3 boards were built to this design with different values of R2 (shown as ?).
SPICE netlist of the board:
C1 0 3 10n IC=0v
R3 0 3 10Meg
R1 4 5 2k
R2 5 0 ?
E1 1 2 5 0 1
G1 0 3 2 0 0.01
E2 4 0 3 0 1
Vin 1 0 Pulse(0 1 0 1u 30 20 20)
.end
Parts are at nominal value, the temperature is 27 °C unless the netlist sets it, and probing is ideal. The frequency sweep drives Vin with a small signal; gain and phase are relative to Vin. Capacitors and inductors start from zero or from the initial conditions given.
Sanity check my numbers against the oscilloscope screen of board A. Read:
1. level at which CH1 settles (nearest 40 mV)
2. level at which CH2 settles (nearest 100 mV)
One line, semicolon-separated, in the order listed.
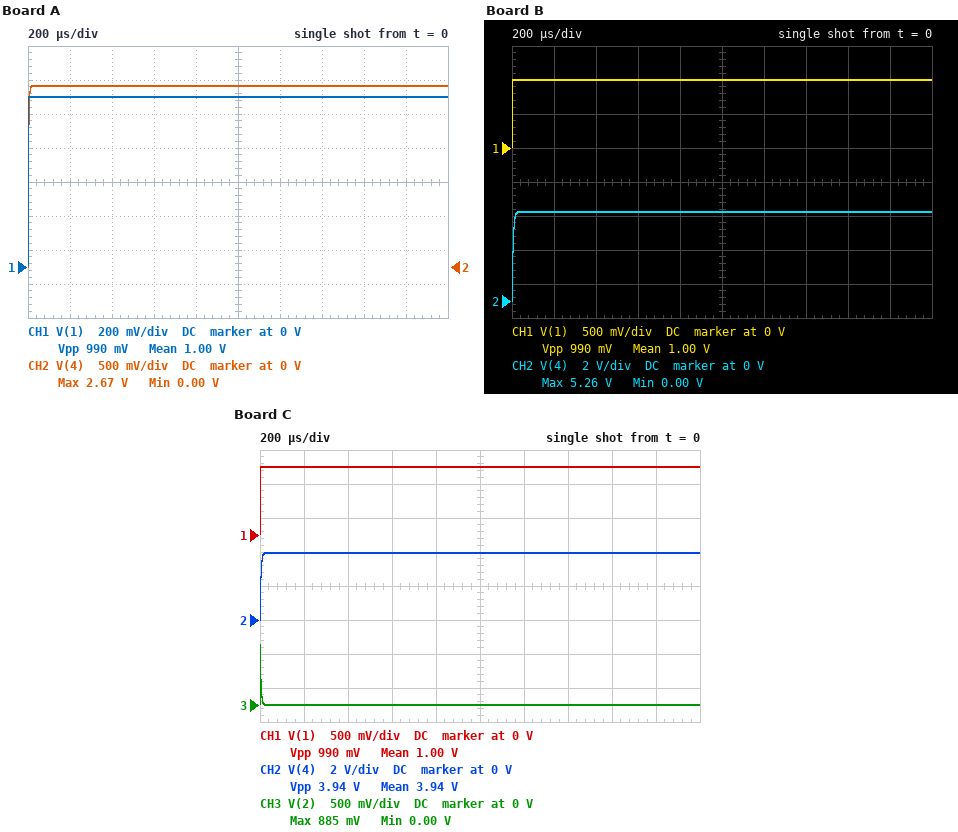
1.00 V; 2.7 V
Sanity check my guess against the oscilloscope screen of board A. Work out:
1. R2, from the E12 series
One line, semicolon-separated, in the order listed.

1.2 kΩ
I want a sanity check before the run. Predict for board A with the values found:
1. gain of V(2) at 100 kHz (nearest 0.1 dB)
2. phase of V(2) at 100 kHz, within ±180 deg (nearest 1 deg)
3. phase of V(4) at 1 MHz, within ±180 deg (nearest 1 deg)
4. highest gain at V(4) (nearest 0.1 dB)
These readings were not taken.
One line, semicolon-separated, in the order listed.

-1.3 dB; 31 deg; -87 deg; 8.5 dB
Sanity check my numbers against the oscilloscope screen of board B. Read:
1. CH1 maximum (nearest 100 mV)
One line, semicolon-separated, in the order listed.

1.0 V
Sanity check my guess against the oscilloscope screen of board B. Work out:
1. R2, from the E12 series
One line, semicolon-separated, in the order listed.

470 Ω
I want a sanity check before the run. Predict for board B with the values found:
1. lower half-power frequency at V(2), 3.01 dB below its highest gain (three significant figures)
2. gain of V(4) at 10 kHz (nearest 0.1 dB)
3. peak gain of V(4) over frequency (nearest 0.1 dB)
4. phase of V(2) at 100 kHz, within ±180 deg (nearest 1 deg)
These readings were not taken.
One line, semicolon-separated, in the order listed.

30.3 kHz; 14.0 dB; 14.4 dB; 17 deg
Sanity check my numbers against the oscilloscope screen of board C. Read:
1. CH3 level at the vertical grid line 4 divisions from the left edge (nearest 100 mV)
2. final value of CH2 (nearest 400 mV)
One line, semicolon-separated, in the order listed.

0 V; 4.0 V
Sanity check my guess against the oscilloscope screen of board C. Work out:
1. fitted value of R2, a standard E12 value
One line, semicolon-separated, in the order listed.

680 Ω
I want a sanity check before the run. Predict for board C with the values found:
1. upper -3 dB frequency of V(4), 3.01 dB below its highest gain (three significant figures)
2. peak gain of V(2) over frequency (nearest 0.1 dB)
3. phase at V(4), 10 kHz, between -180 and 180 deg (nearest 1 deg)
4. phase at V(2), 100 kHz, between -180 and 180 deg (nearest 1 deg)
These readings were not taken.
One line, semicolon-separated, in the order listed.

40.4 kHz; 0 dB; -14 deg; 22 deg
